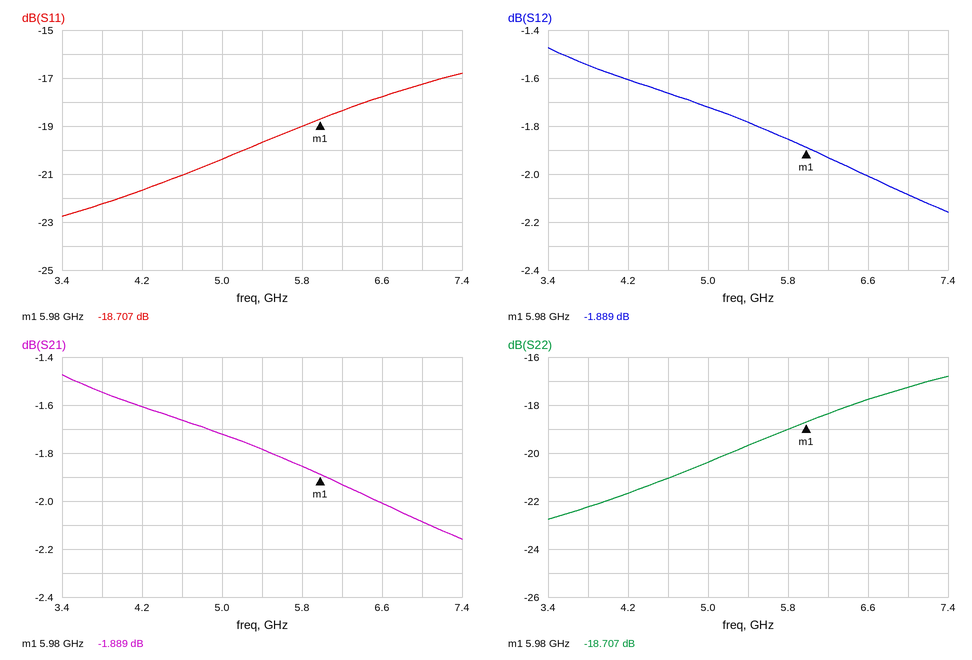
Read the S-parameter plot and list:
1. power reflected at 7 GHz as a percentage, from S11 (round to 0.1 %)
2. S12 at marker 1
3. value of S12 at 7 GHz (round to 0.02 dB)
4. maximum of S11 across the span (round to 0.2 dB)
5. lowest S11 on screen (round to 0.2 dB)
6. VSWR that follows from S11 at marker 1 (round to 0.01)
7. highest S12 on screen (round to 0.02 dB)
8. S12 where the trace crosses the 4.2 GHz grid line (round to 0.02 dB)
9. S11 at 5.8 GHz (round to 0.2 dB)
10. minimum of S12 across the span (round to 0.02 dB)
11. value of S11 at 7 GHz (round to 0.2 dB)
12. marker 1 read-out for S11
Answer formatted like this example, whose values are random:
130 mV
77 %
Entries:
1.9 %
-1.889 dB
-2.08 dB
-16.8 dB
-22.8 dB
1.26
-1.48 dB
-1.60 dB
-19.0 dB
-2.16 dB
-17.2 dB
-18.707 dB
